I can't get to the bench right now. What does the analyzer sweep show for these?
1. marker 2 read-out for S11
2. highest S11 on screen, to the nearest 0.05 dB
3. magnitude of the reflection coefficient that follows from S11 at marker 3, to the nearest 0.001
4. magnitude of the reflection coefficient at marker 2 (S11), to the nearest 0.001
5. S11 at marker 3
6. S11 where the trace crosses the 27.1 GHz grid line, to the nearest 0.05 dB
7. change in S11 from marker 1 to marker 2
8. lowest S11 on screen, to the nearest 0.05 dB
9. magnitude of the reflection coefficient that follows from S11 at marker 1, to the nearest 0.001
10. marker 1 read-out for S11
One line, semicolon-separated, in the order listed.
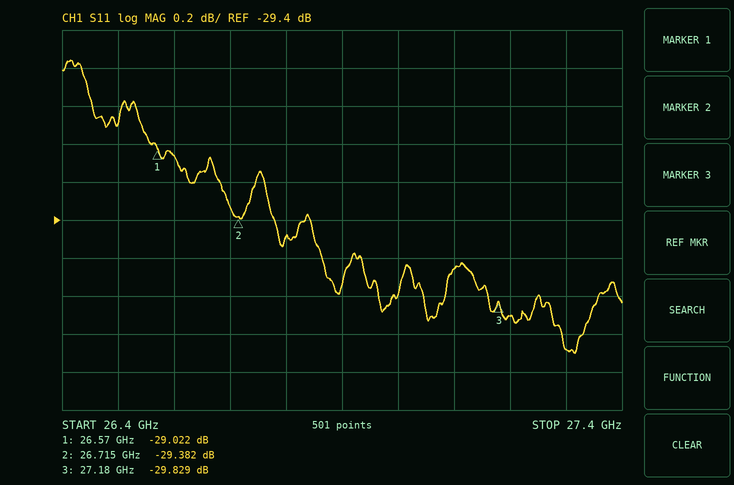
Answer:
-29.382 dB; -28.55 dB; 0.032; 0.034; -29.829 dB; -29.65 dB; -0.360 dB; -30.10 dB; 0.035; -29.022 dB
